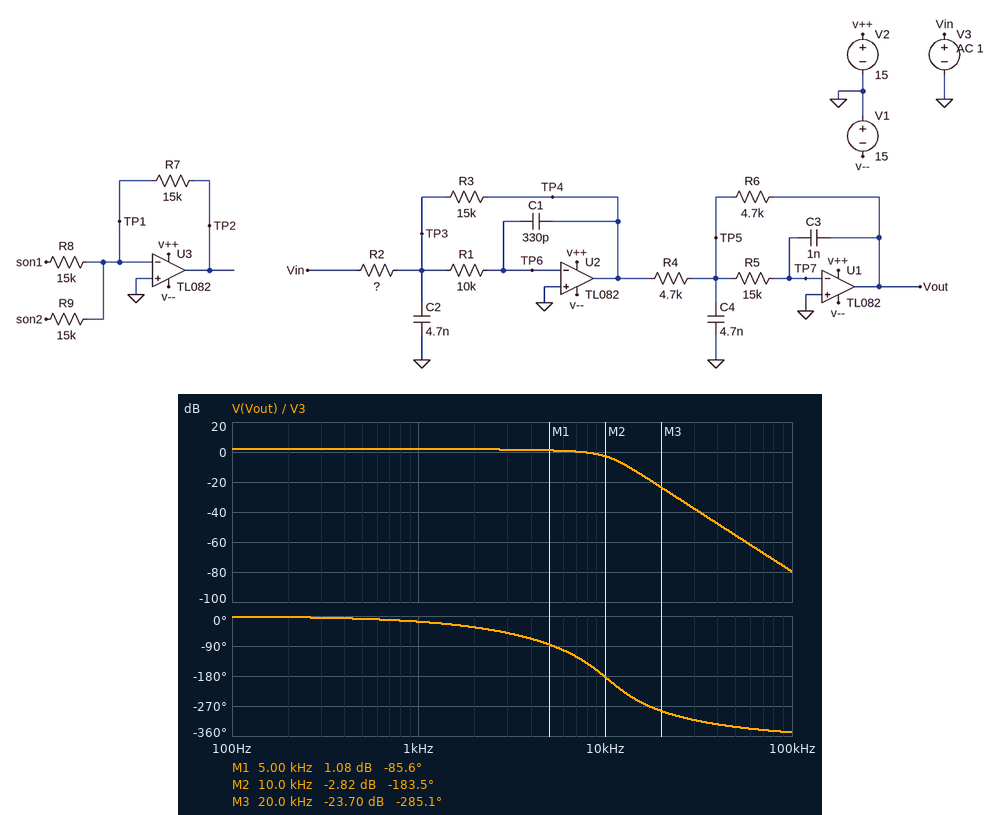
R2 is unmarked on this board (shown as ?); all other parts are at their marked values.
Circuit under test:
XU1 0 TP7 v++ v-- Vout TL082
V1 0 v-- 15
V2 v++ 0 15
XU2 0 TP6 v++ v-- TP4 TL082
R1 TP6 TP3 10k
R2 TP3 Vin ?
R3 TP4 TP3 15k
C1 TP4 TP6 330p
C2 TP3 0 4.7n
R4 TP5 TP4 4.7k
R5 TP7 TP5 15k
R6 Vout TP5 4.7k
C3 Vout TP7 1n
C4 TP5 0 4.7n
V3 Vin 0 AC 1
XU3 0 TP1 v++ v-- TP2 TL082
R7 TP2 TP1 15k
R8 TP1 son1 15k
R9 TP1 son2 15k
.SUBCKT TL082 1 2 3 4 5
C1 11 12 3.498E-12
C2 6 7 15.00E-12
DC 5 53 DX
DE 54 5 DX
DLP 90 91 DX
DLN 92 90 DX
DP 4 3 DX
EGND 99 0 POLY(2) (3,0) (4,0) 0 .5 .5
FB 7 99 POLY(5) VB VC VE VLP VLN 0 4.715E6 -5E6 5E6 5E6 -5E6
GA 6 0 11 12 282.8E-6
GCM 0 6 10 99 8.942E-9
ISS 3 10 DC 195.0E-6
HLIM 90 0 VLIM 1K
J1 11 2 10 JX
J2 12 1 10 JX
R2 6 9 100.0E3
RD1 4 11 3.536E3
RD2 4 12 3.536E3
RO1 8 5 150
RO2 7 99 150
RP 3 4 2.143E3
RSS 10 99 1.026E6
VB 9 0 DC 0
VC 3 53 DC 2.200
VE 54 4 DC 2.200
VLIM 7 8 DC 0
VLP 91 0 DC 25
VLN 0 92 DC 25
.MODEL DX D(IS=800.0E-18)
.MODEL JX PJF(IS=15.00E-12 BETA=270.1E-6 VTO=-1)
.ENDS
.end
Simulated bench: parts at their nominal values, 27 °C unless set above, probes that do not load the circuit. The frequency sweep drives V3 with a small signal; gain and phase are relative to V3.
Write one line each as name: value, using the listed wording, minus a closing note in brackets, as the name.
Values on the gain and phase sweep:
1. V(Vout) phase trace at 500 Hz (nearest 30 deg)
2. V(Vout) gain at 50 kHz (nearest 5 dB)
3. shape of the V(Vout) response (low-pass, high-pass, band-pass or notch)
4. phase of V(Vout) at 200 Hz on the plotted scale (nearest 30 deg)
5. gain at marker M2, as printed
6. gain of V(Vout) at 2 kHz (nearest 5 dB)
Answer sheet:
V(Vout) phase trace at 500 Hz: 0 deg
V(Vout) gain at 50 kHz: -55 dB
shape of the V(Vout) response: low-pass
phase of V(Vout) at 200 Hz on the plotted scale: 0 deg
gain at marker M2, as printed: -2.82 dB
gain of V(Vout) at 2 kHz: 0 dB
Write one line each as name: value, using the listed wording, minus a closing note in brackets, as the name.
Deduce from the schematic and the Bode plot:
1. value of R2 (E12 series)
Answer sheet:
value of R2: 12 kΩ
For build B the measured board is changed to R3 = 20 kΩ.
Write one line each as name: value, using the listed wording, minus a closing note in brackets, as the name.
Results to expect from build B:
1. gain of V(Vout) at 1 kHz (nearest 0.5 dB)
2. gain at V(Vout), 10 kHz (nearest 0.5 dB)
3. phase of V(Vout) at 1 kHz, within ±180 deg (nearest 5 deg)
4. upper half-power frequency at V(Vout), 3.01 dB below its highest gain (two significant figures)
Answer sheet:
gain of V(Vout) at 1 kHz: 4.5 dB
gain at V(Vout), 10 kHz: -2.5 dB
phase of V(Vout) at 1 kHz, within ±180 deg: -20 deg
upper half-power frequency at V(Vout), 3.01 dB below its highest gain: 8.0 kHz
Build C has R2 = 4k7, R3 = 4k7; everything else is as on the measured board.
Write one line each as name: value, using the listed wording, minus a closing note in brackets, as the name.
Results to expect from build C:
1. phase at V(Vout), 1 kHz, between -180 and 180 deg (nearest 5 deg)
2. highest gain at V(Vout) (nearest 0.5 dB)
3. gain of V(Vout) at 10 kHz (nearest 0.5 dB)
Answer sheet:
phase at V(Vout), 1 kHz, between -180 and 180 deg: -15 deg
highest gain at V(Vout): 0 dB
gain of V(Vout) at 10 kHz: -5.5 dB
